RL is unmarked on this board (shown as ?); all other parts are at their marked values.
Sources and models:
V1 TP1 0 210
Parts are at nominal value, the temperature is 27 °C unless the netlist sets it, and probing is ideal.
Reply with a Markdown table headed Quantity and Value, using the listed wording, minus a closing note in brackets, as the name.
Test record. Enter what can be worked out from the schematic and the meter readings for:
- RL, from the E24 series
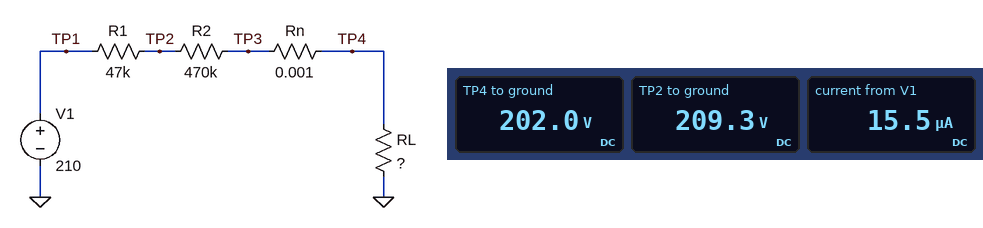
| Quantity | Value |
|---|---|
| RL, from the E24 series | 13 MΩ |
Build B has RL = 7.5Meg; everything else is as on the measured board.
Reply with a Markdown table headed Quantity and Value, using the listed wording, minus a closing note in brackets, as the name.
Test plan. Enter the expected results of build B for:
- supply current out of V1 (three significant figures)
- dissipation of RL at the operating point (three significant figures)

| Quantity | Value |
|---|---|
| supply current out of V1 | 26.2 µA |
| dissipation of RL at the operating point | 5.15 mW |
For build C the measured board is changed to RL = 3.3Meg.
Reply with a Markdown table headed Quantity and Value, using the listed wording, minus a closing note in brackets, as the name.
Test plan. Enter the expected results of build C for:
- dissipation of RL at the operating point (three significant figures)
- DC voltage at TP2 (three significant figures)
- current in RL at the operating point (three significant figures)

| Quantity | Value |
|---|---|
| dissipation of RL at the operating point | 9.99 mW |
| DC voltage at TP2 | 207 V |
| current in RL at the operating point | 55.0 µA |
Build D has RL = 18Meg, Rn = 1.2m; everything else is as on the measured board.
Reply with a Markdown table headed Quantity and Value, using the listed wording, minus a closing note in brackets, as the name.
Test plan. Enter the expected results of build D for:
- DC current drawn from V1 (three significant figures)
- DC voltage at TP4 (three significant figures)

| Quantity | Value |
|---|---|
| DC current drawn from V1 | 11.3 µA |
| DC voltage at TP4 | 204 V |
